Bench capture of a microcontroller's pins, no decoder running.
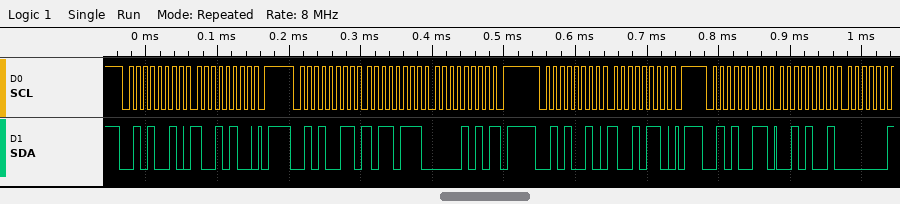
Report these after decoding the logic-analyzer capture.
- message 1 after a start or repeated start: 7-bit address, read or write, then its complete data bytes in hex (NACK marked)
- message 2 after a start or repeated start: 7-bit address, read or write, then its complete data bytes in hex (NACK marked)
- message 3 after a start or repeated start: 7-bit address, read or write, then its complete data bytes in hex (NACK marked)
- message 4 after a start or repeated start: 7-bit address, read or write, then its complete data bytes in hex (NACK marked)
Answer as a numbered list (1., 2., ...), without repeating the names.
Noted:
1. 0x29 write: 94
2. 0x29 read: B7 0A NACK
3. 0x29 write: 96
4. 0x29 read: 29
